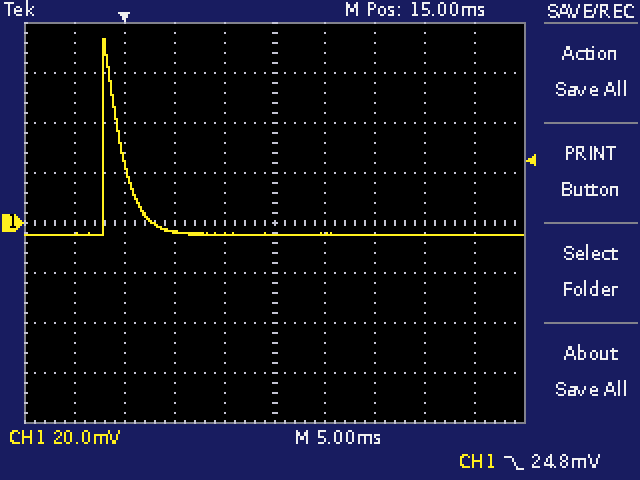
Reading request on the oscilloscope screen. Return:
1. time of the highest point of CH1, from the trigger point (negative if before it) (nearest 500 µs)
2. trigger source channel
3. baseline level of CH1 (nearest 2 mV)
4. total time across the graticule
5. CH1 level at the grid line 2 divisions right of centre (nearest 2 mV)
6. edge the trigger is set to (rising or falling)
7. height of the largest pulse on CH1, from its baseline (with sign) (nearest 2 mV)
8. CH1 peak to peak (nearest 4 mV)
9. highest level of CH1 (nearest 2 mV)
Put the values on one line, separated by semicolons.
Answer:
-2.0 ms; CH1; -4 mV; 50 ms; -4 mV; falling; +78 mV; 80 mV; 74 mV
